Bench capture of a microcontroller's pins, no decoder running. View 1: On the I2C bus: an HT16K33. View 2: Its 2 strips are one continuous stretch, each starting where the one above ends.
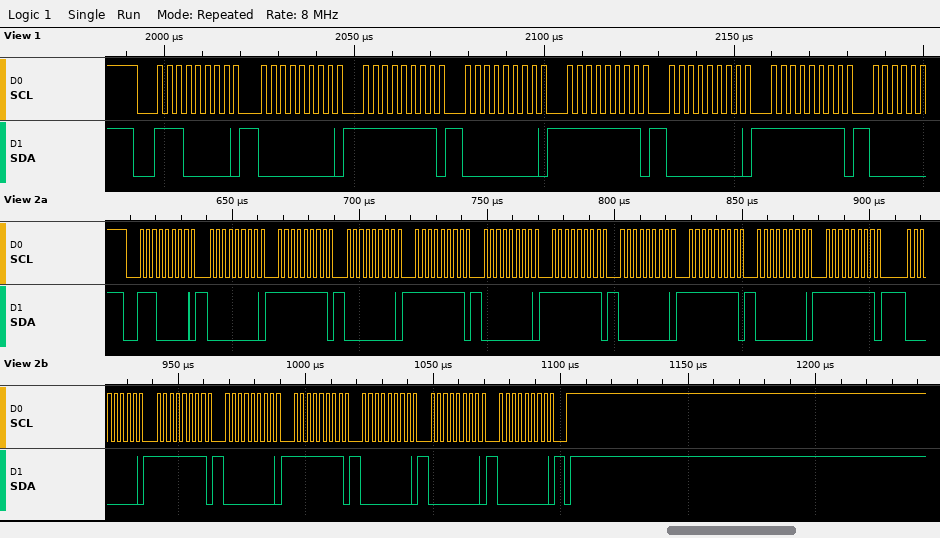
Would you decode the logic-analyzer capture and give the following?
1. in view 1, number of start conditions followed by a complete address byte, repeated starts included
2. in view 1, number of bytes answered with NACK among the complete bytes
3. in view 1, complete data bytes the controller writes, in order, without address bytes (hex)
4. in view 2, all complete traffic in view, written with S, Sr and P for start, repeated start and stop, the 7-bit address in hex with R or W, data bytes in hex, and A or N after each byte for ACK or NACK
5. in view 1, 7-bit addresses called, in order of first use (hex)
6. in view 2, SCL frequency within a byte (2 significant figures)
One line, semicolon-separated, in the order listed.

1; 0; 00 FF 00 FF 00 FF; S 70W A 00 A FF A 00 A FF A 00 A FF A 00 A FF A 00 A FF A 00 A FF A 00 A FF A 00 A 00 A 00 A P; 0x70; 400 kHz
